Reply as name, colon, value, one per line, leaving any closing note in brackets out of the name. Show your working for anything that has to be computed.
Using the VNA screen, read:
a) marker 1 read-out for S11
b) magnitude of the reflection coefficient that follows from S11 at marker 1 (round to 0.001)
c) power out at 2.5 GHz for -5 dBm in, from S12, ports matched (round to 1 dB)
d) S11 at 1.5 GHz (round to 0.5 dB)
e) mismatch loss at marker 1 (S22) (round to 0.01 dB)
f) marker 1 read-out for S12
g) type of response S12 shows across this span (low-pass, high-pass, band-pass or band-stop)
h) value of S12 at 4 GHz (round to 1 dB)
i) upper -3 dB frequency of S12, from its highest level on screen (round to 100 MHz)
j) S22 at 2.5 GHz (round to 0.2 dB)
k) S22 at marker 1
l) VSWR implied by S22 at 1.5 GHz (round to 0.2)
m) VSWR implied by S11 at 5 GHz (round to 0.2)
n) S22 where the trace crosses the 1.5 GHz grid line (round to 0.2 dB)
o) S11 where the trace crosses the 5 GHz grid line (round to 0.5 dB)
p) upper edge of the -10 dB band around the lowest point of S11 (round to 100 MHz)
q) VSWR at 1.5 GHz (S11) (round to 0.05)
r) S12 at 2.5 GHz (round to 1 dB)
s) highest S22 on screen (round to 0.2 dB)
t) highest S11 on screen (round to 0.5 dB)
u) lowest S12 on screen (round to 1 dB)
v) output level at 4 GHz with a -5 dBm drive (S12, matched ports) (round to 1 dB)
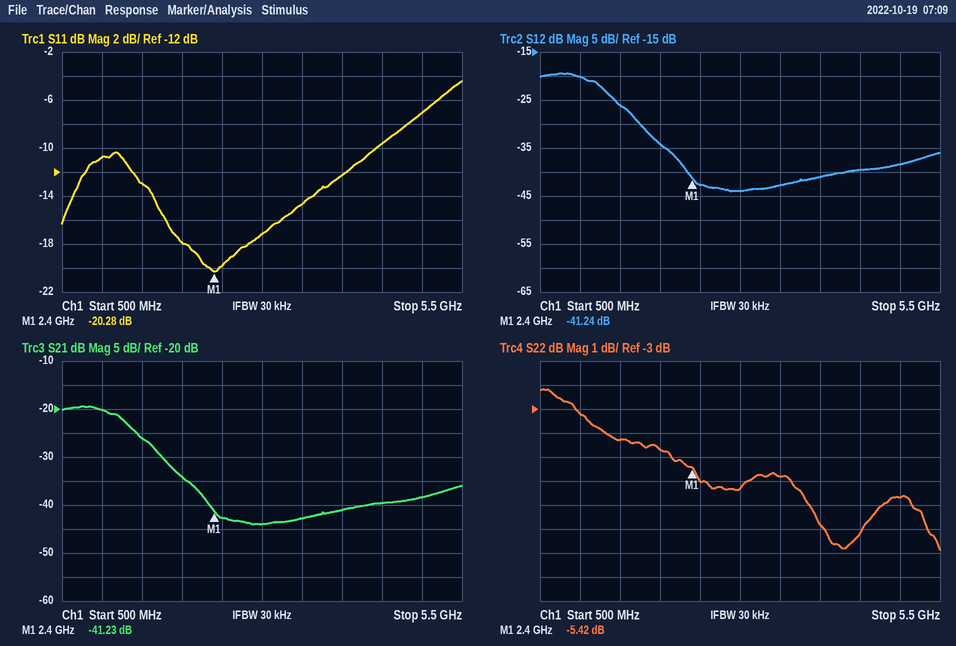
marker 1 read-out for S11: -20.28 dB
magnitude of the reflection coefficient that follows from S11 at marker 1: 10^(-20.28/20) ≈ 0.097
power out at 2.5 GHz for -5 dBm in, from S12, ports matched: -5 dBm + (-43 dB) = -48 dBm
S11 at 1.5 GHz: -13.0 dB
mismatch loss at marker 1 (S22): −10 log10(1 − 10^(-5.42/10)) ≈ 1.47 dB
marker 1 read-out for S12: -41.24 dB
type of response S12 shows across this span: low-pass
value of S12 at 4 GHz: -41 dB
upper -3 dB frequency of S12, from its highest level on screen: 1.3 GHz
S22 at 2.5 GHz: -6.0 dB
S22 at marker 1: -5.42 dB
VSWR implied by S22 at 1.5 GHz: |Γ| = 10^(-4.2/20) = 0.6166; VSWR = (1 + 0.6166)/(1 − 0.6166) ≈ 4.2
VSWR implied by S11 at 5 GHz: |Γ| = 10^(-7/20) = 0.4467; VSWR = (1 + 0.4467)/(1 − 0.4467) ≈ 2.6
S22 where the trace crosses the 1.5 GHz grid line: -4.2 dB
S11 where the trace crosses the 5 GHz grid line: -7.0 dB
upper edge of the -10 dB band around the lowest point of S11: 4.4 GHz
VSWR at 1.5 GHz (S11): |Γ| = 10^(-13/20) = 0.2239; VSWR = (1 + 0.2239)/(1 − 0.2239) ≈ 1.58, so 1.60 to the nearest 0.05
S12 at 2.5 GHz: -43 dB
highest S22 on screen: -2.2 dB
highest S11 on screen: -4.5 dB
lowest S12 on screen: -44 dB
output level at 4 GHz with a -5 dBm drive (S12, matched ports): -5 dBm + (-41 dB) = -46 dBm
